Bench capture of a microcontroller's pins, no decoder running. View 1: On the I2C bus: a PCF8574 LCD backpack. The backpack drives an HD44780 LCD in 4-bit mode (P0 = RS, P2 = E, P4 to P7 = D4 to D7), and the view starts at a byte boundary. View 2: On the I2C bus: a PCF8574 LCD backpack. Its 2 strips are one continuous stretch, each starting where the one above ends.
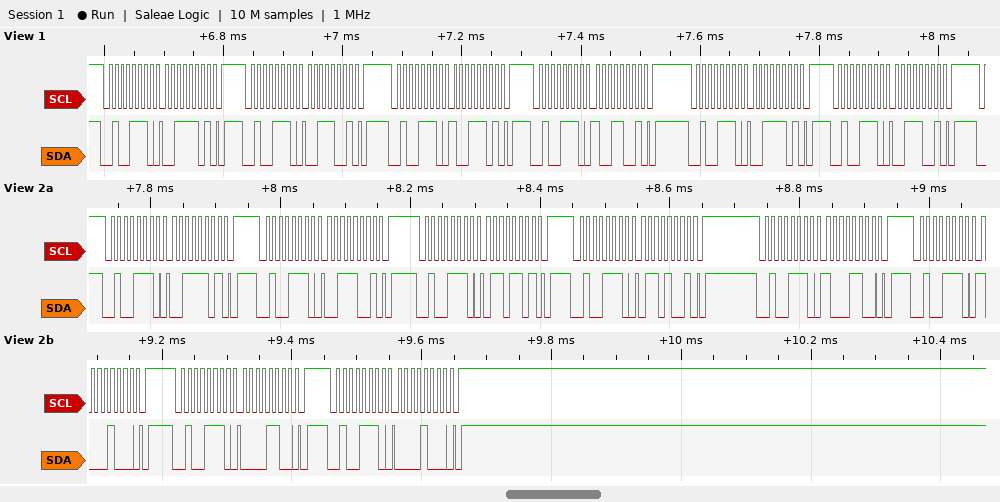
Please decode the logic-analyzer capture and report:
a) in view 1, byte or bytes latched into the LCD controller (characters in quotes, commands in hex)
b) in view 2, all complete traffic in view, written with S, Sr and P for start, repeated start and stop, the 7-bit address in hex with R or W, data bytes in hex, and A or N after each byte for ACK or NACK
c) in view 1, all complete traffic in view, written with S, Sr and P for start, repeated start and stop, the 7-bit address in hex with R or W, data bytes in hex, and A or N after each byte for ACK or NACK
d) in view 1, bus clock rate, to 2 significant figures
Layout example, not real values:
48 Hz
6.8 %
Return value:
'9'
S 27W A 3D A P S 27W A 39 A P S 27W A 6D A P S 27W A 69 A P S 27W A 8C A P S 27W A 88 A P S 27W A 0C A P S 27W A 08 A P
S 27W A 3D A P S 27W A 39 A P S 27W A 9D A P S 27W A 99 A P S 27W A 3D A P S 27W A 39 A P
100 kHz
